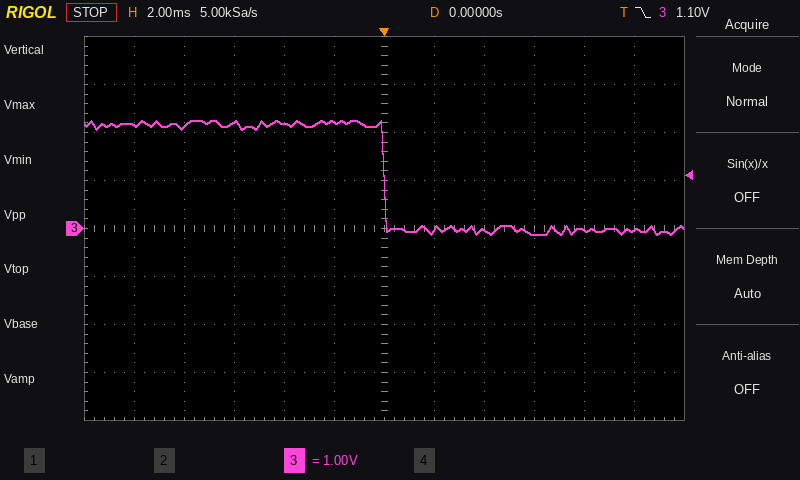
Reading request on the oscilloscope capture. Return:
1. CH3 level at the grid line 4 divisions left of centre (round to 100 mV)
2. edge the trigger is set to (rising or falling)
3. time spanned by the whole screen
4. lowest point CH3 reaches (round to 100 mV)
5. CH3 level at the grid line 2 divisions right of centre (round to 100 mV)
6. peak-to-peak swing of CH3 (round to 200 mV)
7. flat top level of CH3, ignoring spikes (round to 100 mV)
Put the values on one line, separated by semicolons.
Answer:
2.1 V; falling; 24 ms; -100 mV; 0.0 V; 2.4 V; 2.2 V
